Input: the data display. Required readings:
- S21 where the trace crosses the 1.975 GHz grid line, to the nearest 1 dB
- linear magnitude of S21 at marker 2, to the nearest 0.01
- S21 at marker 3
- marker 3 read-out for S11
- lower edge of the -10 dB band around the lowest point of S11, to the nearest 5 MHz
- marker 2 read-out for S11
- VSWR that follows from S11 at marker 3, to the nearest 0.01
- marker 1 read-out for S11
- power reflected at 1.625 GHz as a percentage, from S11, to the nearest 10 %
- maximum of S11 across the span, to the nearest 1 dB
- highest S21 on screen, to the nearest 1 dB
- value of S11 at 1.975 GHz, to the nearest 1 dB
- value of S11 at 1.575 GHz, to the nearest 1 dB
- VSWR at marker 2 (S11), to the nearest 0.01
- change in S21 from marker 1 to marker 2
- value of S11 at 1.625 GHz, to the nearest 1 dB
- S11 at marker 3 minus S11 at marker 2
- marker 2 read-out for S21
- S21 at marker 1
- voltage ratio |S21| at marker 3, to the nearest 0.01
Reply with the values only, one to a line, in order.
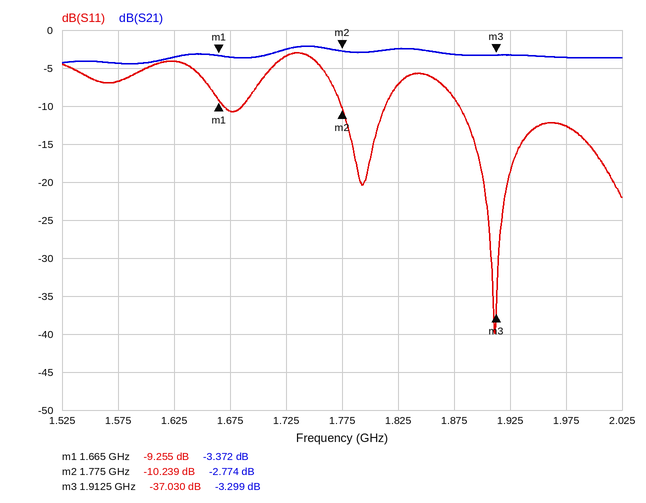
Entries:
-4 dB
0.73
-3.299 dB
-37.030 dB
1.880 GHz
-10.239 dB
1.03
-9.255 dB
40 %
-3 dB
-2 dB
-13 dB
-7 dB
1.89
0.598 dB
-4 dB
-26.791 dB
-2.774 dB
-3.372 dB
0.68
